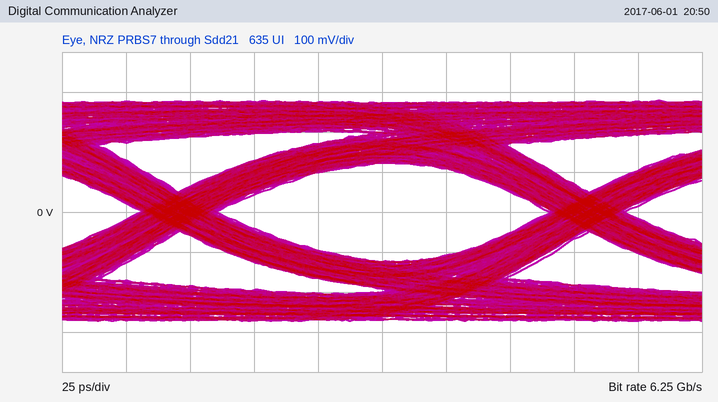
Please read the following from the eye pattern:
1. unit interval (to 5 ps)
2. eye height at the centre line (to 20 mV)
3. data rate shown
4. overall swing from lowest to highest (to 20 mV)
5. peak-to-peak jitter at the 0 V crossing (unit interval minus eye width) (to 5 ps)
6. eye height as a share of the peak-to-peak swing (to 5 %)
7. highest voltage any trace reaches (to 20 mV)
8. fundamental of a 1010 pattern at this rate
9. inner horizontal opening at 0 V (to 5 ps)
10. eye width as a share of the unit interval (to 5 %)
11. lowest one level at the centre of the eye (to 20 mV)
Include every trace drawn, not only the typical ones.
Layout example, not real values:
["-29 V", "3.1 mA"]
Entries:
["160 ps", "240 mV", "6.25 Gb/s", "560 mV", "30 ps", "45 %", "280 mV", "3.125 GHz", "130 ps", "80 %", "120 mV"]
